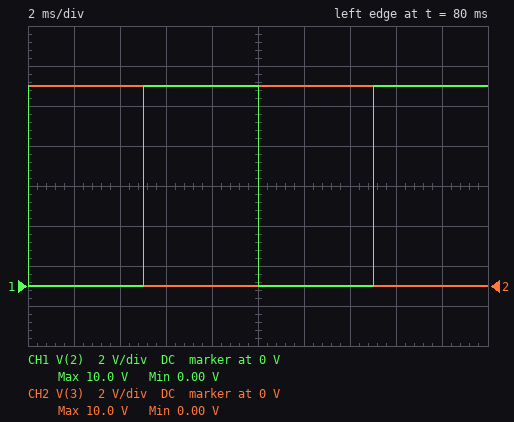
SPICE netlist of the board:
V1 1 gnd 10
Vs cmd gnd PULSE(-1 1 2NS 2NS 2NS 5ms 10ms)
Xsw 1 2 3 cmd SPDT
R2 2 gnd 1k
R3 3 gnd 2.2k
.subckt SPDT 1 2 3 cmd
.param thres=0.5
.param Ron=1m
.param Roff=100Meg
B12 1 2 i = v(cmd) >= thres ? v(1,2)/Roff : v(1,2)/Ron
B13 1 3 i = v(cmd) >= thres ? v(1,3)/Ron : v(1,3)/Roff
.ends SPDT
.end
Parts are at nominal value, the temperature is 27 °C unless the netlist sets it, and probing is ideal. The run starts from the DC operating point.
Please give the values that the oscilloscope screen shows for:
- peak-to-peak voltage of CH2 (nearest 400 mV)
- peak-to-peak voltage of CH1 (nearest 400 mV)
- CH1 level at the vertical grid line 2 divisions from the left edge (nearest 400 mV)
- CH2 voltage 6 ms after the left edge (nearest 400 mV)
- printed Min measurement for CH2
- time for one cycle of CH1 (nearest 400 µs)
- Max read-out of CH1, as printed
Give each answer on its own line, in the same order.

10.0 V
10.0 V
0 V
0 V
0.00 V
10.0 ms
10.0 V
